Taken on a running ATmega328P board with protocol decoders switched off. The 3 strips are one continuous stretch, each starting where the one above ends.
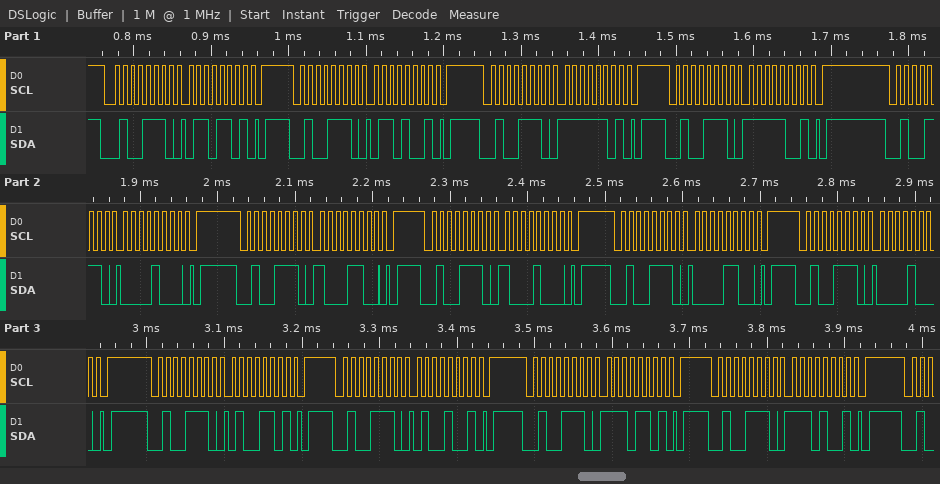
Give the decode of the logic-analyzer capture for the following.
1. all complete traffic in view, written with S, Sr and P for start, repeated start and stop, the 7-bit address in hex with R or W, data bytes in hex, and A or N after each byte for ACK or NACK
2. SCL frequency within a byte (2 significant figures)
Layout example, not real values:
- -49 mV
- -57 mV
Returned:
- S 27W A 6D A P S 27W A 69 A P S 27W A FD A P S 27W A F9 A P S 27W A 08 A P S 27W A 8C A P S 27W A 88 A P S 27W A 0C A P S 27W A 08 A P S 27W A 4D A P S 27W A 49 A P S 27W A ED A P S 27W A E9 A P
- 100 kHz
